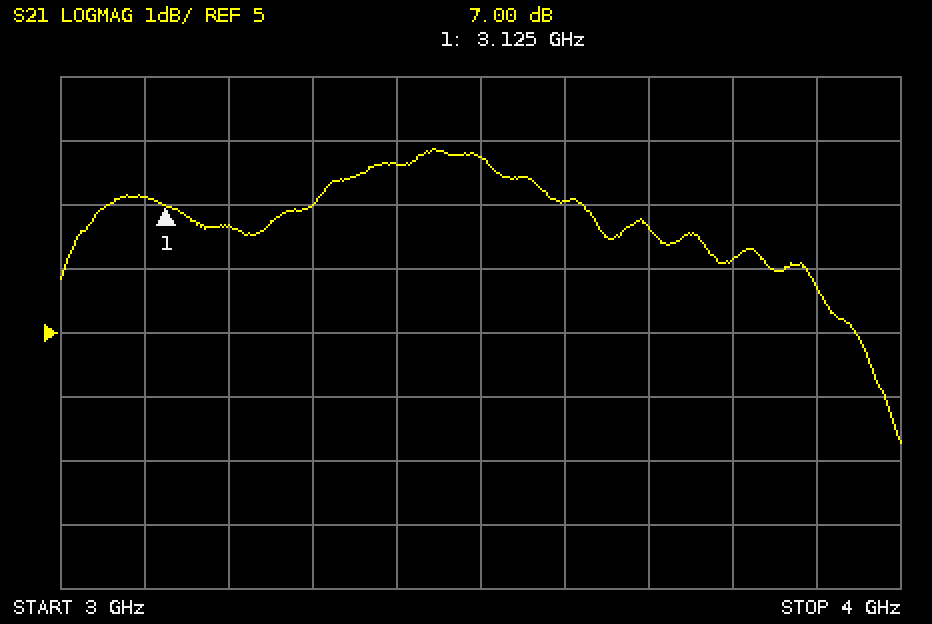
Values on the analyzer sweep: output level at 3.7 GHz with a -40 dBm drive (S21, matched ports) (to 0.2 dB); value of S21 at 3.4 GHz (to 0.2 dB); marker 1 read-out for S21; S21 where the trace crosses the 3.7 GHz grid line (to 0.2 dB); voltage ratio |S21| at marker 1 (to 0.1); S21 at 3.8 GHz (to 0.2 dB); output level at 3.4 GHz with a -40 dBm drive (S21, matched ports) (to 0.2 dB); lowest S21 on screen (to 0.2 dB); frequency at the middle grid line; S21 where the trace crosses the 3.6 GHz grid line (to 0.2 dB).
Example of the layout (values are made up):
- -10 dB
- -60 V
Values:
- -33.4 dBm
- 7.6 dB
- 7.00 dB
- 6.6 dB
- 2.2
- 6.2 dB
- -32.4 dBm
- 3.2 dB
- 3.5 GHz
- 7.0 dB
